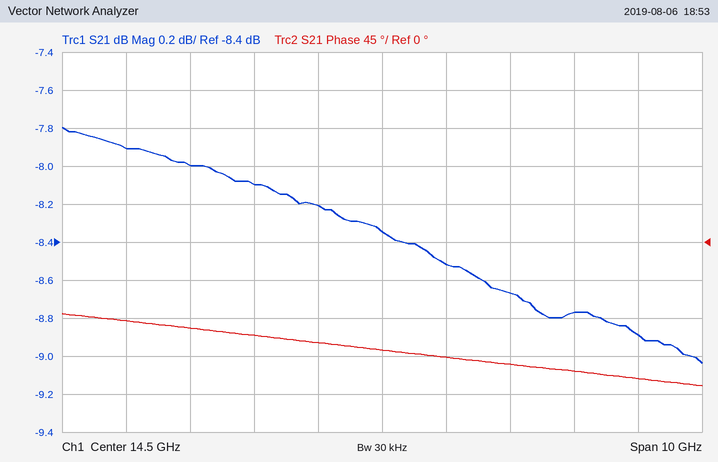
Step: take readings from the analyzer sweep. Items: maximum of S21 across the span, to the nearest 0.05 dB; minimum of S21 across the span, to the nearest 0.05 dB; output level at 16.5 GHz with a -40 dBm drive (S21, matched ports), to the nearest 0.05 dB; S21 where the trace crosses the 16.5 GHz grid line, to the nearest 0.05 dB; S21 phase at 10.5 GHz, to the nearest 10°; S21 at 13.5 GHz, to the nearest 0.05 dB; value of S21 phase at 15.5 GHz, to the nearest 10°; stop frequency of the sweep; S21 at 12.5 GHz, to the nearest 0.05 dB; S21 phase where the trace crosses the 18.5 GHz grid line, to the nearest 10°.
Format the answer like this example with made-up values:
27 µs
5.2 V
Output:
-7.80 dB
-9.05 dB
-48.65 dBm
-8.65 dB
-90°
-8.20 dB
-140°
19.5 GHz
-8.10 dB
-160°
